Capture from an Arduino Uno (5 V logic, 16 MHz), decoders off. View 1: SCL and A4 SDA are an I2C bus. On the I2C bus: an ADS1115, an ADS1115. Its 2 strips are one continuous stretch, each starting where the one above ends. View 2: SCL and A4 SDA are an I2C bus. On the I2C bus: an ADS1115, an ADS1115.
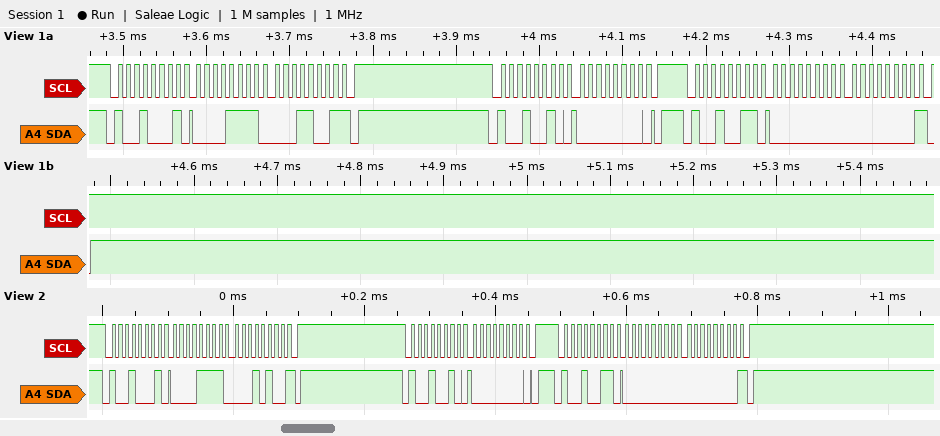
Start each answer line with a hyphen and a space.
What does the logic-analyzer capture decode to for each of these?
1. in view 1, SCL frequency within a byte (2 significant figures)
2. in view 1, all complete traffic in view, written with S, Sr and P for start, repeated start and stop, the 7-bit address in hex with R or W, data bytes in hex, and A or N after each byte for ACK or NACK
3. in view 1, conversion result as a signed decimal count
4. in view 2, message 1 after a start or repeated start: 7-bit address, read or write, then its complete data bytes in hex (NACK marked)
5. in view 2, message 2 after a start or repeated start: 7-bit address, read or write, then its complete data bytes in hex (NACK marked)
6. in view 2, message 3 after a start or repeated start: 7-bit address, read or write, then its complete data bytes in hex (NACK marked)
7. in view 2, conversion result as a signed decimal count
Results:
- 100 kHz
- S 48R A 0F A 19 N P S 49W A 00 A P S 49R A 00 A 00 N P
- 0
- 0x48 read: 0F 14 NACK
- 0x49 write: 00
- 0x49 read: 00 00 NACK
- 0
